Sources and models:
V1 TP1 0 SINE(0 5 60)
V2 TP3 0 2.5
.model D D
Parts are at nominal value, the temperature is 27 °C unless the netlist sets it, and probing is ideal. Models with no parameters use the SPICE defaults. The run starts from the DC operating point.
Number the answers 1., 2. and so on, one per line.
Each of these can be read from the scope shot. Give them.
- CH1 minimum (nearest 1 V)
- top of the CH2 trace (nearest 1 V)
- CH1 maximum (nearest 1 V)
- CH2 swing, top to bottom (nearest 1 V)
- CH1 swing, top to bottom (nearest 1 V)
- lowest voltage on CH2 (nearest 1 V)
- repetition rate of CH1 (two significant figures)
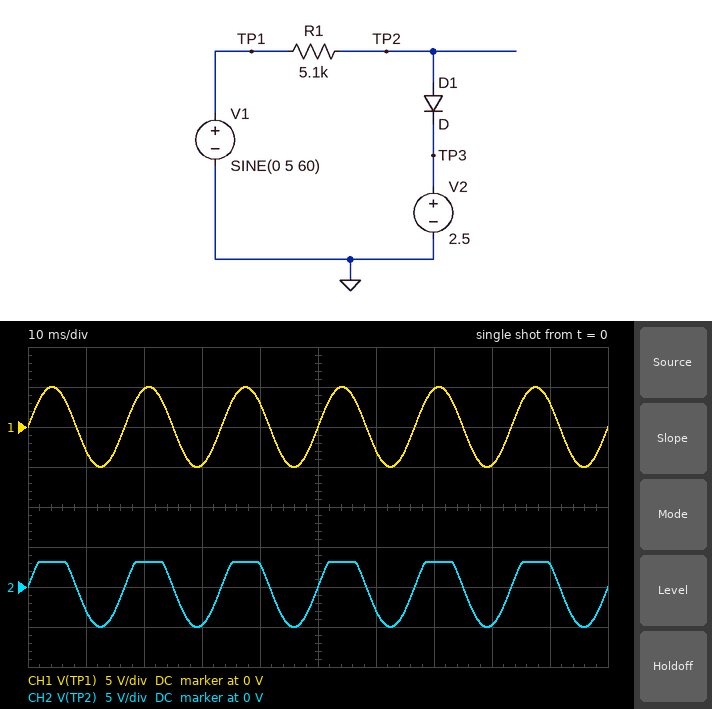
1. -5 V
2. 3 V
3. 5 V
4. 8 V
5. 10 V
6. -5 V
7. 60 Hz
